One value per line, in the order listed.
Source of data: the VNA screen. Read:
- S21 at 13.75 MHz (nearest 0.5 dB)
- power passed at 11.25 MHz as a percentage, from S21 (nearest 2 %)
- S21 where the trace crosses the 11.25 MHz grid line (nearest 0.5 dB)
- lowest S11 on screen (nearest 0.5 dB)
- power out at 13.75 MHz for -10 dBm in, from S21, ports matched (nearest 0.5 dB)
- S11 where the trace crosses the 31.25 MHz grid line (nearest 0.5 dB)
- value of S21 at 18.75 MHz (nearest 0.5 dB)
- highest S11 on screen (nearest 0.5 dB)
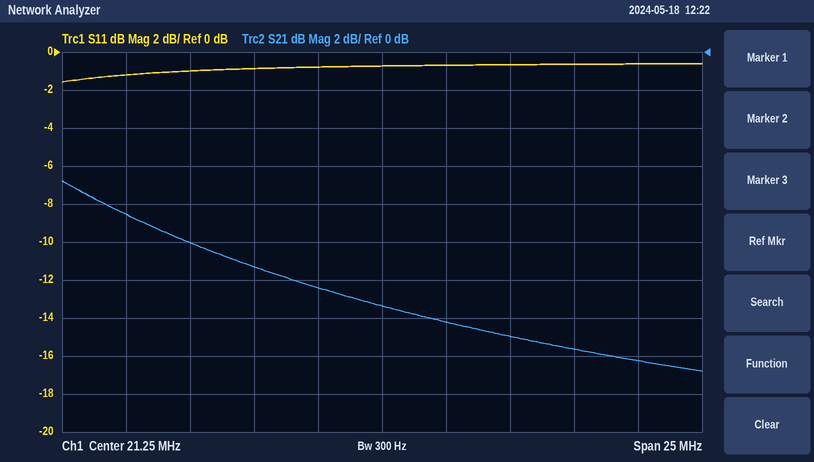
-10.0 dB
14 %
-8.5 dB
-1.5 dB
-20.0 dBm
-0.5 dB
-12.5 dB
-0.5 dB
